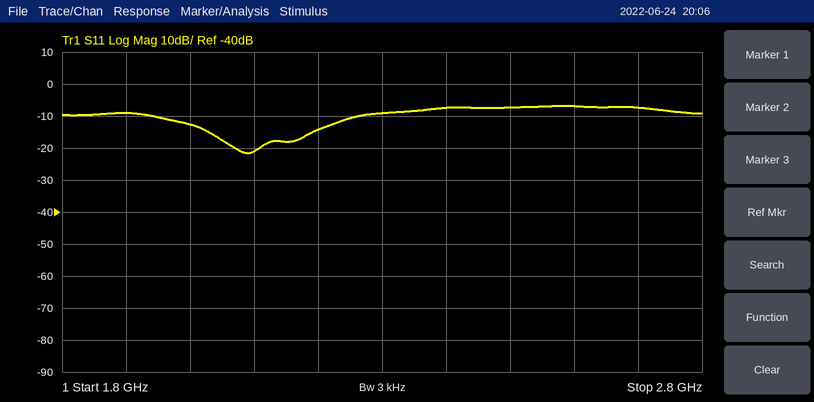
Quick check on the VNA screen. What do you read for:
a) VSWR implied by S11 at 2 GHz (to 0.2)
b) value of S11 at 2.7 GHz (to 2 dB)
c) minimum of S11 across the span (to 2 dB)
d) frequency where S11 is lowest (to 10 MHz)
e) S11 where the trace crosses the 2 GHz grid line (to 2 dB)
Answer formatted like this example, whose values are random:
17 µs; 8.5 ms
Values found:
1.6; -8 dB; -22 dB; 2.09 GHz; -12 dB
